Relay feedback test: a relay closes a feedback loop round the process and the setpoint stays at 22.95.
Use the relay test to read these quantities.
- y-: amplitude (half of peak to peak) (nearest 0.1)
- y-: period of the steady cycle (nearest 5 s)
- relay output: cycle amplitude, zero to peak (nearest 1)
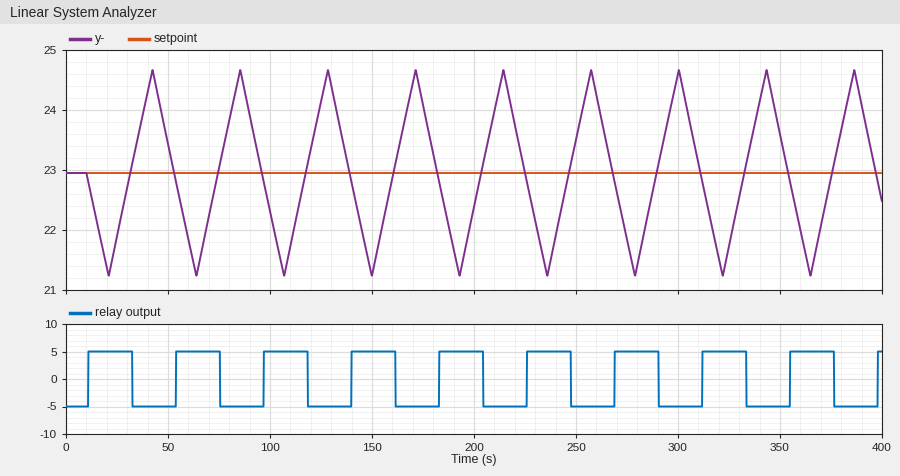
1.7
45 s
5
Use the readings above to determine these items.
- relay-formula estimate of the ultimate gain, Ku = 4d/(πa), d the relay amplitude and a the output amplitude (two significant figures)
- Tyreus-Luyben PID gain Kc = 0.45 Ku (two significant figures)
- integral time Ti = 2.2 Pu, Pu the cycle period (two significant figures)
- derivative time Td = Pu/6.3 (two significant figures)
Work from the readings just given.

3.7
1.7
99 s
7.1 s
